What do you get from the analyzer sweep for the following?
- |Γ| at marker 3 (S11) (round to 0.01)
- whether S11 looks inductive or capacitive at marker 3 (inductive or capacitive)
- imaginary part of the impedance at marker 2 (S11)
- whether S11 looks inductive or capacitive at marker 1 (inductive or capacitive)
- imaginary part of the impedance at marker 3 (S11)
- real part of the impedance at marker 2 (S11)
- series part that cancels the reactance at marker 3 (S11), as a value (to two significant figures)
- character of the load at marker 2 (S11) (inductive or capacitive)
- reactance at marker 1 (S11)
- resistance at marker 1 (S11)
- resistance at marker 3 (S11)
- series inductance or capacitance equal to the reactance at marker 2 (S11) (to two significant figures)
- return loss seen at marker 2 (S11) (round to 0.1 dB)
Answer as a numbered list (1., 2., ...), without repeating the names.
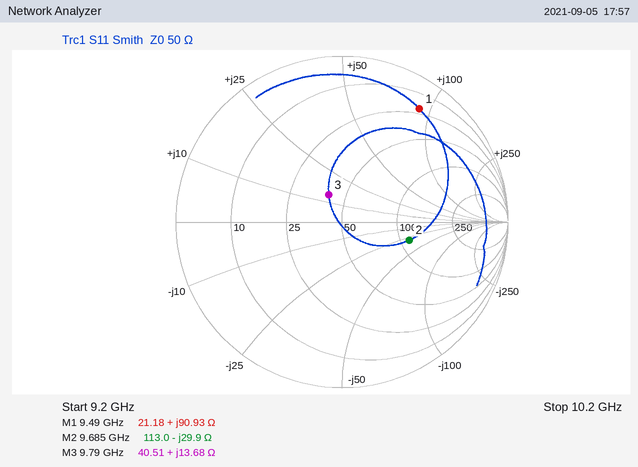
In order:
1. 0.18
2. inductive
3. -29.9 Ω
4. inductive
5. +13.68 Ω
6. 113.0 Ω
7. 1.2 pF
8. capacitive
9. +90.93 Ω
10. 21.18 Ω
11. 40.51 Ω
12. 550 fF
13. 7.5 dB
